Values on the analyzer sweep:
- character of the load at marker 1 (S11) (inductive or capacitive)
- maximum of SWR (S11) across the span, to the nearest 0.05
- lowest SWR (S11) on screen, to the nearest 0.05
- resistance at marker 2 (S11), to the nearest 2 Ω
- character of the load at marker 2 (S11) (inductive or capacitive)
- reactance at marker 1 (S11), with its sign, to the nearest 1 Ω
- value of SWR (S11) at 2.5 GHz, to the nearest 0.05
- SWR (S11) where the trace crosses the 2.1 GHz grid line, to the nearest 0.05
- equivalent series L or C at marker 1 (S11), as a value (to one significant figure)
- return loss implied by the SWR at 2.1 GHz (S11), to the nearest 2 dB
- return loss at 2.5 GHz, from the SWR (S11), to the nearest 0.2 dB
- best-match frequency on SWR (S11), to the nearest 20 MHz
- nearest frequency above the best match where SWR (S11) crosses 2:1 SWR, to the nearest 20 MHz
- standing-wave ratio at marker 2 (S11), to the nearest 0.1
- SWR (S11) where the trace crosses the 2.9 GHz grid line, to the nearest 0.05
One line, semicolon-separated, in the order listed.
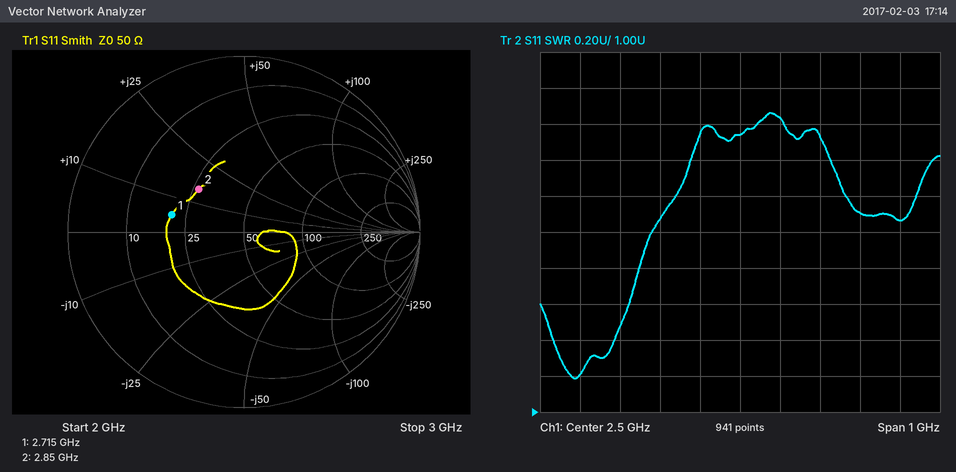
inductive; 2.65; 1.20; 26 Ω; inductive; +5 Ω; 2.55; 1.20; 300 pH; 20 dB; 7.2 dB; 2.08 GHz; 2.28 GHz; 2.1; 2.05
